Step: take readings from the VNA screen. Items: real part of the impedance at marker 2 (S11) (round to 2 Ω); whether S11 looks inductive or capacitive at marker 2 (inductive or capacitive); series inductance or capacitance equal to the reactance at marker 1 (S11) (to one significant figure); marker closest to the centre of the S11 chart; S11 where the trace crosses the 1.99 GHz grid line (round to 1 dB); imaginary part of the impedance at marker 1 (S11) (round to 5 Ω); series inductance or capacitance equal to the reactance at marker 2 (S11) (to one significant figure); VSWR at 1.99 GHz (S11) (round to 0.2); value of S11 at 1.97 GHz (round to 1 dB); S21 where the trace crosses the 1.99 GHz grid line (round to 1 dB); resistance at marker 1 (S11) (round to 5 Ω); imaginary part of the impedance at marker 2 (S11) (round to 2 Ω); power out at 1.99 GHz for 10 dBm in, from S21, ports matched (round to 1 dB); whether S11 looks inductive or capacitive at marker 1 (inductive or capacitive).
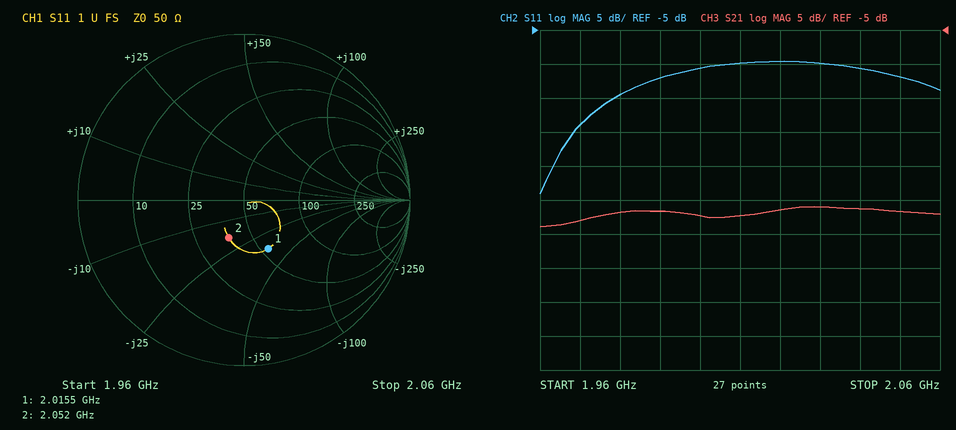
38 Ω
capacitive
2 pF
marker 2
-12 dB
-35 Ω
4 pF
1.6
-19 dB
-32 dB
55 Ω
-18 Ω
-22 dBm
capacitive
